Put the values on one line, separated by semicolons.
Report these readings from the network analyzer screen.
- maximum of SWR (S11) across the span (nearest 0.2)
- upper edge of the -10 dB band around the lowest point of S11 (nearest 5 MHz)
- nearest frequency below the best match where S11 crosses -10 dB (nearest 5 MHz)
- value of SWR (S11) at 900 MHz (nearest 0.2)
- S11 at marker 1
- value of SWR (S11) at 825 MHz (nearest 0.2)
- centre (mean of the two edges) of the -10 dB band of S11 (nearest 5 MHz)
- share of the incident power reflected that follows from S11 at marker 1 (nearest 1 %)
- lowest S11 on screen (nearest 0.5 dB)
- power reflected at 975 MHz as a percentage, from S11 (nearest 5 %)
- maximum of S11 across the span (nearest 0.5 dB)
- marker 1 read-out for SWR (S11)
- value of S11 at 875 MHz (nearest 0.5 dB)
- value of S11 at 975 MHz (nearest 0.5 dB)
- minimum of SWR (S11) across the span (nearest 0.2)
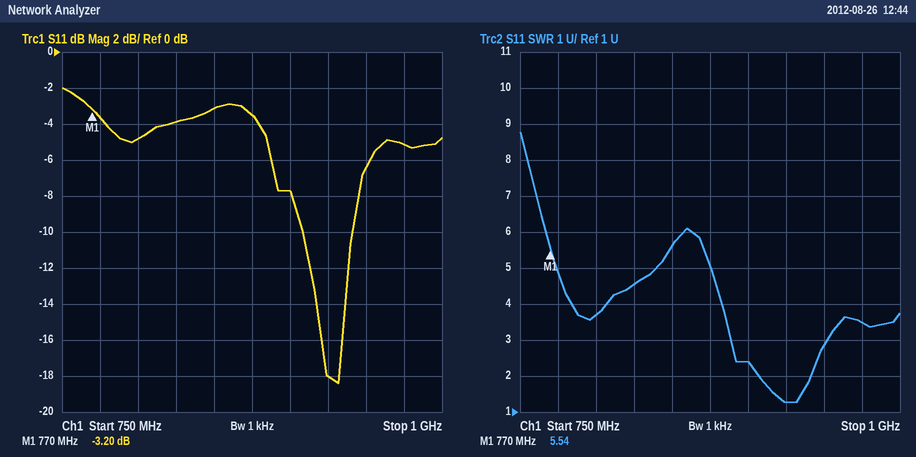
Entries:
8.8; 940 MHz; 910 MHz; 2.4; -3.20 dB; 4.6; 925 MHz; 48 %; -18.5 dB; 30 %; -2.0 dB; 5.54; -3.5 dB; -5.0 dB; 1.2
